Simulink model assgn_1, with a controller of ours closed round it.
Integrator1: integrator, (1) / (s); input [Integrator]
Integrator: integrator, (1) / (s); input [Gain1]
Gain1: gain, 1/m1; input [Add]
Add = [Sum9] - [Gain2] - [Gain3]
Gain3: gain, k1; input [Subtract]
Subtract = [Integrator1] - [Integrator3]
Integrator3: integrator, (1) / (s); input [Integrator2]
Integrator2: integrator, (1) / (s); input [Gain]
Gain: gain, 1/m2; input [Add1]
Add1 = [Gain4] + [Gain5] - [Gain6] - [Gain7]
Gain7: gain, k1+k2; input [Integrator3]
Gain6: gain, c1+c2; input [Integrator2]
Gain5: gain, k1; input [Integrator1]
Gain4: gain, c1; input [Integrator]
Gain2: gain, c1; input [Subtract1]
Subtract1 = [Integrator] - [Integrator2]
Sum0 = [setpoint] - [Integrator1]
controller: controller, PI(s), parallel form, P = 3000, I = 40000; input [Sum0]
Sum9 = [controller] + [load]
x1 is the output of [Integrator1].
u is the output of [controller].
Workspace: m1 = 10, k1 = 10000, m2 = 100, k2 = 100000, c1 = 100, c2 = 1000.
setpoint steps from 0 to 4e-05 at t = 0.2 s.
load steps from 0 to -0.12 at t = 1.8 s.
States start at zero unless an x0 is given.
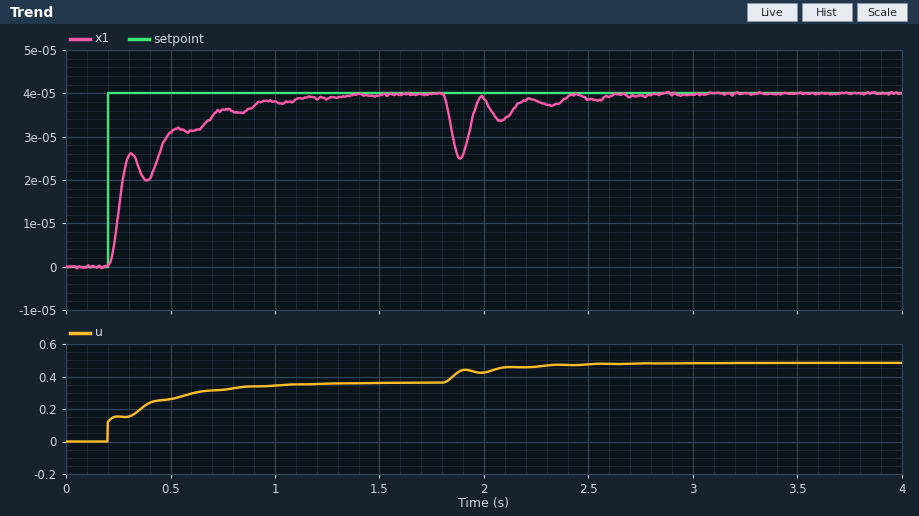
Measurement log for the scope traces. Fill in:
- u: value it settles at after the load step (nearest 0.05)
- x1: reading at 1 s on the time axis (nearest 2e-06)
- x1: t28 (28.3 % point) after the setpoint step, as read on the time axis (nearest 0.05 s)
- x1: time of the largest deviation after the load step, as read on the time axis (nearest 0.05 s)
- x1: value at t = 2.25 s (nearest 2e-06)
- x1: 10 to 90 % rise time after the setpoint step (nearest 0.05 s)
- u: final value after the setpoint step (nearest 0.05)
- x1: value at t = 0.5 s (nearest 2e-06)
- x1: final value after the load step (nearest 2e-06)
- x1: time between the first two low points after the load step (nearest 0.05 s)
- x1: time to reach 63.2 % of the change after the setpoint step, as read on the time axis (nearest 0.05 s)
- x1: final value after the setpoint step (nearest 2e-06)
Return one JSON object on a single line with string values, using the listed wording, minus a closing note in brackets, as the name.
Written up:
{"u: value it settles at after the load step": "0.50", "x1: reading at 1 s on the time axis": "0.000038", "x1: t28 (28.3 % point) after the setpoint step, as read on the time axis": "0.25 s", "x1: time of the largest deviation after the load step, as read on the time axis": "1.90 s", "x1: value at t = 2.25 s": "0.000038", "x1: 10 to 90 % rise time after the setpoint step": "0.50 s", "u: final value after the setpoint step": "0.35", "x1: value at t = 0.5 s": "0.000032", "x1: final value after the load step": "0.000040", "x1: time between the first two low points after the load step": "0.20 s", "x1: time to reach 63.2 % of the change after the setpoint step, as read on the time axis": "0.30 s", "x1: final value after the setpoint step": "0.000040"}
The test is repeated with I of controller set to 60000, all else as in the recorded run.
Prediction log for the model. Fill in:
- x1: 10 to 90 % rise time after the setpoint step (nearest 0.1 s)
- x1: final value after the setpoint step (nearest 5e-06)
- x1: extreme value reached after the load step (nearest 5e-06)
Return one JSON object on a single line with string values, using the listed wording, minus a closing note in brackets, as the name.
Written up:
{"x1: 10 to 90 % rise time after the setpoint step": "0.3 s", "x1: final value after the setpoint step": "0.000040", "x1: extreme value reached after the load step": "0.000025"}
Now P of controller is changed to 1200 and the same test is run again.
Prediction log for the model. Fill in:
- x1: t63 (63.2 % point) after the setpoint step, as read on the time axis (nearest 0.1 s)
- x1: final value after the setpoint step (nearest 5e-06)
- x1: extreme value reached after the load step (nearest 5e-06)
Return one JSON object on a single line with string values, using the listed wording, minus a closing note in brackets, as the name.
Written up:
{"x1: t63 (63.2 % point) after the setpoint step, as read on the time axis": "0.5 s", "x1: final value after the setpoint step": "0.000040", "x1: extreme value reached after the load step": "0.000025"}
